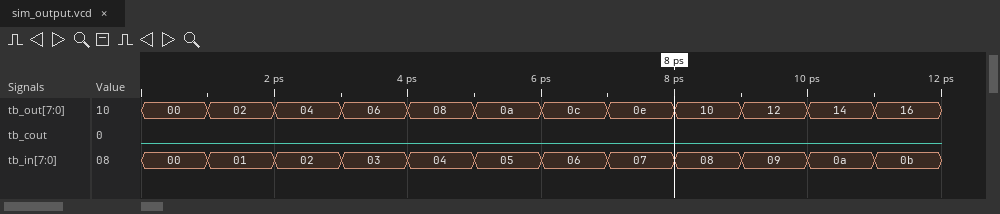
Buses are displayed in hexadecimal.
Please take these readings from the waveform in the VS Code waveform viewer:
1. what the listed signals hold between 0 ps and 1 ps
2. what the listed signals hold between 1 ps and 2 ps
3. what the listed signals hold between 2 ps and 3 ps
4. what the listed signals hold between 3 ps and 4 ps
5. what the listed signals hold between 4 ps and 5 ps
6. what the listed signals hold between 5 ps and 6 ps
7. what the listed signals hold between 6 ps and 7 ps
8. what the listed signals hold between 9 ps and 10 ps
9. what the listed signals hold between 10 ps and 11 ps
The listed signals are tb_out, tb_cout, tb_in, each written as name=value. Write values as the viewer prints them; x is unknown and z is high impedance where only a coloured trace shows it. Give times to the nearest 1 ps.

tb_out=00, tb_cout=0, tb_in=00
tb_out=02, tb_cout=0, tb_in=01
tb_out=04, tb_cout=0, tb_in=02
tb_out=06, tb_cout=0, tb_in=03
tb_out=08, tb_cout=0, tb_in=04
tb_out=0a, tb_cout=0, tb_in=05
tb_out=0c, tb_cout=0, tb_in=06
tb_out=12, tb_cout=0, tb_in=09
tb_out=14, tb_cout=0, tb_in=0a
